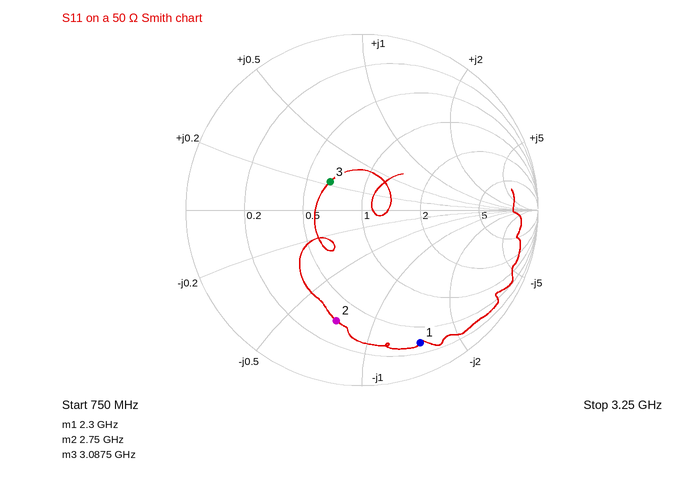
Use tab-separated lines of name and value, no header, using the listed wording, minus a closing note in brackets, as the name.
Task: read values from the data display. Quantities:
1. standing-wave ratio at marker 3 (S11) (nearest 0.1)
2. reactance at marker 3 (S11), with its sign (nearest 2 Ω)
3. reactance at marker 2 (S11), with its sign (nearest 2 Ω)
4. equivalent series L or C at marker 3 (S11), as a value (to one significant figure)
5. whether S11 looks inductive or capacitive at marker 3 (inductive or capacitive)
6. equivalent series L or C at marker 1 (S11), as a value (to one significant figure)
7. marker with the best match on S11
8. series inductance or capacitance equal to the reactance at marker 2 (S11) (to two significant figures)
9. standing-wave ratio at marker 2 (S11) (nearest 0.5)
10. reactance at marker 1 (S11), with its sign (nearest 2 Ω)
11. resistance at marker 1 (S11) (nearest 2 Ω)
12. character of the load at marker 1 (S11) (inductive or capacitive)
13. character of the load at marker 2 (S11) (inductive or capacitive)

standing-wave ratio at marker 3 (S11)	1.6
reactance at marker 3 (S11), with its sign	+12 Ω
reactance at marker 2 (S11), with its sign	-36 Ω
equivalent series L or C at marker 3 (S11), as a value	600 pH
whether S11 looks inductive or capacitive at marker 3	inductive
equivalent series L or C at marker 1 (S11), as a value	900 fF
marker with the best match on S11	marker 3
series inductance or capacitance equal to the reactance at marker 2 (S11)	1.6 pF
standing-wave ratio at marker 2 (S11)	4.5
reactance at marker 1 (S11), with its sign	-74 Ω
resistance at marker 1 (S11)	16 Ω
character of the load at marker 1 (S11)	capacitive
character of the load at marker 2 (S11)	capacitive
